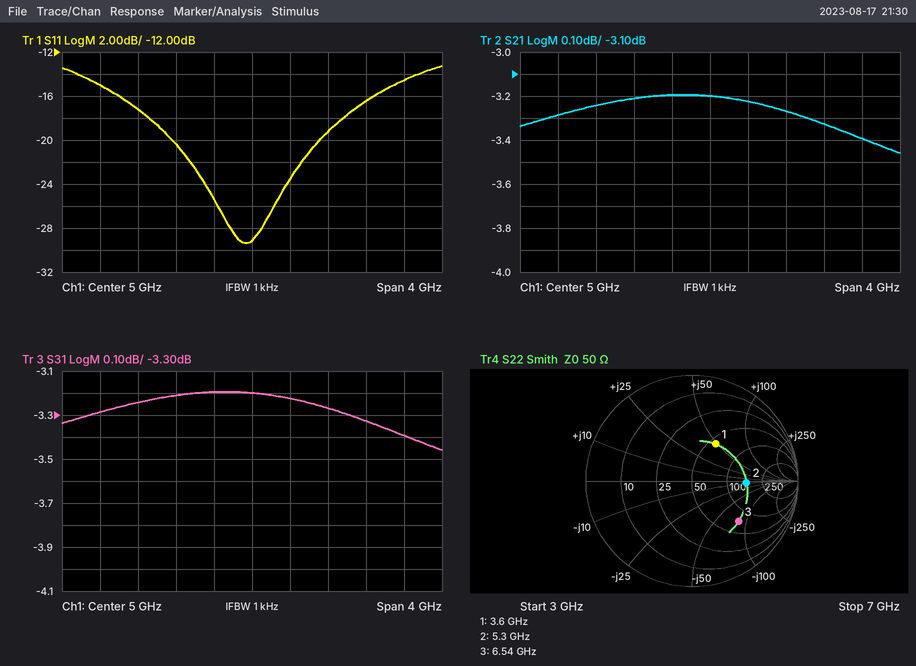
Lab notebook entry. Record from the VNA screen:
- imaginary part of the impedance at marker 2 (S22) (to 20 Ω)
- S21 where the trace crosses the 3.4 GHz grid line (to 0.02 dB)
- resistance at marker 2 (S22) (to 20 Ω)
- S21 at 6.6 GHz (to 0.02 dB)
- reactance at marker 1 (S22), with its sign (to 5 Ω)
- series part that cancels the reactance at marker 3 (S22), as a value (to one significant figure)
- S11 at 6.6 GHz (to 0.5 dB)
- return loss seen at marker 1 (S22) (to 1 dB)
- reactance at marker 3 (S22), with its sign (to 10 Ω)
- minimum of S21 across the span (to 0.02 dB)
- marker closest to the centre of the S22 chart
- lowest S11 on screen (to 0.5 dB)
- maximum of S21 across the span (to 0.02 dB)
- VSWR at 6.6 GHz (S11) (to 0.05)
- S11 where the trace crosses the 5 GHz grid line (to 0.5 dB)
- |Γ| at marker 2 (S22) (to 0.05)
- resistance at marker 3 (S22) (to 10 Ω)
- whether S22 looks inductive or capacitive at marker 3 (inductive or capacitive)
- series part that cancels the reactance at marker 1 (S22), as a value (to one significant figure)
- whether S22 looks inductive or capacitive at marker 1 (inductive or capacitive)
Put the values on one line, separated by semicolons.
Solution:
0 Ω; -3.28 dB; 160 Ω; -3.40 dB; +50 Ω; 2 nH; -14.5 dB; 8 dB; -80 Ω; -3.46 dB; marker 1; -29.5 dB; -3.20 dB; 1.45; -29.0 dB; 0.50; 70 Ω; capacitive; 900 fF; inductive
